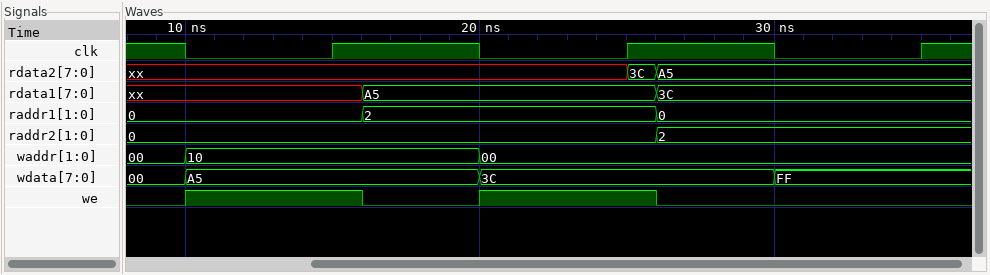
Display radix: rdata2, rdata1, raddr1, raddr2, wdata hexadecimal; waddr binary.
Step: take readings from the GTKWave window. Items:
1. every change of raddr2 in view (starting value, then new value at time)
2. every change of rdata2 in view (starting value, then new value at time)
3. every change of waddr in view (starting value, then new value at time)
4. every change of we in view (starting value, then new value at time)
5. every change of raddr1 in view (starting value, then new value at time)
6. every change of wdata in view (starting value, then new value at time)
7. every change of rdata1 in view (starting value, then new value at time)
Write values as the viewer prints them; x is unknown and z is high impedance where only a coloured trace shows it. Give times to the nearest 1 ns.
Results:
0, 2 at 26 ns
xx, 3C at 25 ns, A5 at 26 ns
00, 10 at 10 ns, 00 at 20 ns
0, 1 at 10 ns, 0 at 16 ns, 1 at 20 ns, 0 at 26 ns
0, 2 at 16 ns, 0 at 26 ns
00, A5 at 10 ns, 3C at 20 ns, FF at 30 ns
xx, A5 at 16 ns, 3C at 26 ns
